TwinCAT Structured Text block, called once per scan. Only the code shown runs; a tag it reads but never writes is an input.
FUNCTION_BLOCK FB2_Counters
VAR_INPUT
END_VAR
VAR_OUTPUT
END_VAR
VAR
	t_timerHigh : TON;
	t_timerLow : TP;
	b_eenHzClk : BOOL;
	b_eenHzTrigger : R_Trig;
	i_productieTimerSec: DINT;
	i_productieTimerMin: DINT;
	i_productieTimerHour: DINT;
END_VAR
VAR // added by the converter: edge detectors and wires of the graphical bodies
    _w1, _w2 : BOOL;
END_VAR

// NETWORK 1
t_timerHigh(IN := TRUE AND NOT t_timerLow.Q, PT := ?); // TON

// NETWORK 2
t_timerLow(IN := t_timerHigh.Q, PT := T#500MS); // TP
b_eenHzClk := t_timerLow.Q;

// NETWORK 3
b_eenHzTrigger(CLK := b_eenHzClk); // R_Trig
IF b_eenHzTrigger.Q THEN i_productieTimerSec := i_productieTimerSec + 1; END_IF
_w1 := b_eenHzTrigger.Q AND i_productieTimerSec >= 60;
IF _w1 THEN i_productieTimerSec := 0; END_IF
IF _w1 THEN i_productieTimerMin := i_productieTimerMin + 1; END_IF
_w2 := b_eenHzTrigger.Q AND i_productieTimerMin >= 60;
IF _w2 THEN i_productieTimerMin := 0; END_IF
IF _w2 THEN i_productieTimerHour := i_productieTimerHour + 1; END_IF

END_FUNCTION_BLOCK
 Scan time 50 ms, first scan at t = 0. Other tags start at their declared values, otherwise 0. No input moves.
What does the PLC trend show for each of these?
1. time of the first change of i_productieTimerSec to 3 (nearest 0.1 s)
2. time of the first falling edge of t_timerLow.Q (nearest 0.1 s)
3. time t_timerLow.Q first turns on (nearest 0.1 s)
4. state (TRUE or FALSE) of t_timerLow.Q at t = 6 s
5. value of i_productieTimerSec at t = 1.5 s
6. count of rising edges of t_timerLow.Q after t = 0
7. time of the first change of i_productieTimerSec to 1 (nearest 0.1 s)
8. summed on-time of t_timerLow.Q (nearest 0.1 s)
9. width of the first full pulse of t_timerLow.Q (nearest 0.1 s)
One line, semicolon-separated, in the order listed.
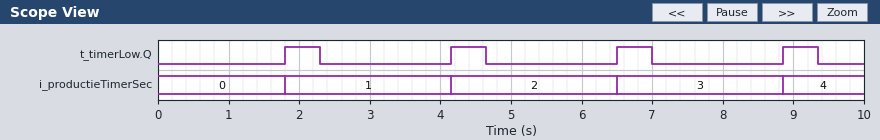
6.5 s; 2.3 s; 1.8 s; FALSE; 0; 4; 1.8 s; 2.0 s; 0.5 s
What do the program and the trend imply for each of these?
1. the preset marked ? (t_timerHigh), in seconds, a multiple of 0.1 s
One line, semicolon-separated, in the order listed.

1.8 s
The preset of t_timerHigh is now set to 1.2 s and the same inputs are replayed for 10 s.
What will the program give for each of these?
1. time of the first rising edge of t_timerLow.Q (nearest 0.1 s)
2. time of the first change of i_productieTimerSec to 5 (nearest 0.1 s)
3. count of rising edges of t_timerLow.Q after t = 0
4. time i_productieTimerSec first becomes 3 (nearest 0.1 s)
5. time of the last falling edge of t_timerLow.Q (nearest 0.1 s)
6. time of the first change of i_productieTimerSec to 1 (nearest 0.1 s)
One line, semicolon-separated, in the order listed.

1.2 s; 8.2 s; 6; 4.7 s; 8.7 s; 1.2 s
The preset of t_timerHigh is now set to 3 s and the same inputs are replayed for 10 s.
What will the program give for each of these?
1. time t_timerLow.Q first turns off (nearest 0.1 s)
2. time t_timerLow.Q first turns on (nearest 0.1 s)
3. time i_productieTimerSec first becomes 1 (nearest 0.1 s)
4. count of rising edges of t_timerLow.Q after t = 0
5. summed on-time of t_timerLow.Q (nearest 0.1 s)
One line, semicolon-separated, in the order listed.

3.5 s; 3.0 s; 3.0 s; 2; 1.0 s
